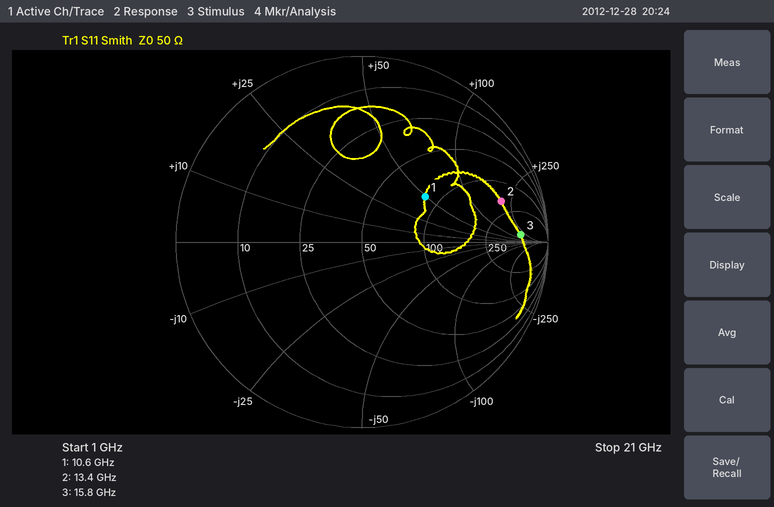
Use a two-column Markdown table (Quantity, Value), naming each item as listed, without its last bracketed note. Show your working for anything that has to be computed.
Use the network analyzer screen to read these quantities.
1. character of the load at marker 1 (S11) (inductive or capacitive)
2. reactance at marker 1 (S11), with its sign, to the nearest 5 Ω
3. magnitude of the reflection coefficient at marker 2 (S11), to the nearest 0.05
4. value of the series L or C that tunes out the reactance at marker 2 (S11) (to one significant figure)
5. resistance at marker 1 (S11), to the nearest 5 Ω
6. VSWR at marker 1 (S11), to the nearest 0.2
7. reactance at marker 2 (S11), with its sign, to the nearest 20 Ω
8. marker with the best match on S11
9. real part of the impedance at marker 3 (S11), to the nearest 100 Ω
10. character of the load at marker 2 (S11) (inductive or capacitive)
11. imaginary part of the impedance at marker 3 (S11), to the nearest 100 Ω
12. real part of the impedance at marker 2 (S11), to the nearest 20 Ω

| Quantity | Value |
|---|---|
| character of the load at marker 1 (S11) | inductive |
| reactance at marker 1 (S11), with its sign, to the nearest 5 Ω | +50 Ω |
| magnitude of the reflection coefficient at marker 2 (S11), to the nearest 0.05 | 0.80 |
| value of the series L or C that tunes out the reactance at marker 2 (S11) | C = 1/(2π × 13.4 GHz × 200 Ω) ≈ 59.4 fF, so 60 fF to one significant figure |
| resistance at marker 1 (S11), to the nearest 5 Ω | 85 Ω |
| VSWR at marker 1 (S11), to the nearest 0.2 | 2.4 |
| reactance at marker 2 (S11), with its sign, to the nearest 20 Ω | +200 Ω |
| marker with the best match on S11 | marker 1 |
| real part of the impedance at marker 3 (S11), to the nearest 100 Ω | 600 Ω |
| character of the load at marker 2 (S11) | inductive |
| imaginary part of the impedance at marker 3 (S11), to the nearest 100 Ω | +200 Ω |
| real part of the impedance at marker 2 (S11), to the nearest 20 Ω | 180 Ω |
